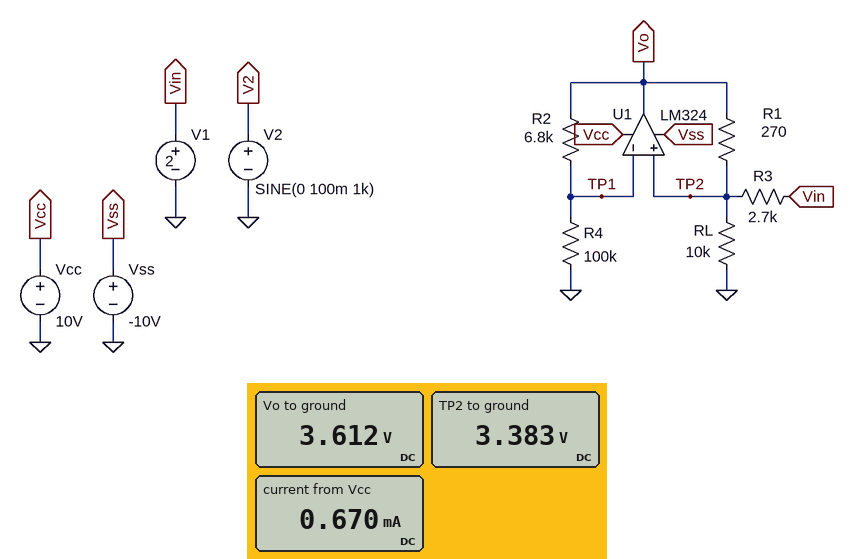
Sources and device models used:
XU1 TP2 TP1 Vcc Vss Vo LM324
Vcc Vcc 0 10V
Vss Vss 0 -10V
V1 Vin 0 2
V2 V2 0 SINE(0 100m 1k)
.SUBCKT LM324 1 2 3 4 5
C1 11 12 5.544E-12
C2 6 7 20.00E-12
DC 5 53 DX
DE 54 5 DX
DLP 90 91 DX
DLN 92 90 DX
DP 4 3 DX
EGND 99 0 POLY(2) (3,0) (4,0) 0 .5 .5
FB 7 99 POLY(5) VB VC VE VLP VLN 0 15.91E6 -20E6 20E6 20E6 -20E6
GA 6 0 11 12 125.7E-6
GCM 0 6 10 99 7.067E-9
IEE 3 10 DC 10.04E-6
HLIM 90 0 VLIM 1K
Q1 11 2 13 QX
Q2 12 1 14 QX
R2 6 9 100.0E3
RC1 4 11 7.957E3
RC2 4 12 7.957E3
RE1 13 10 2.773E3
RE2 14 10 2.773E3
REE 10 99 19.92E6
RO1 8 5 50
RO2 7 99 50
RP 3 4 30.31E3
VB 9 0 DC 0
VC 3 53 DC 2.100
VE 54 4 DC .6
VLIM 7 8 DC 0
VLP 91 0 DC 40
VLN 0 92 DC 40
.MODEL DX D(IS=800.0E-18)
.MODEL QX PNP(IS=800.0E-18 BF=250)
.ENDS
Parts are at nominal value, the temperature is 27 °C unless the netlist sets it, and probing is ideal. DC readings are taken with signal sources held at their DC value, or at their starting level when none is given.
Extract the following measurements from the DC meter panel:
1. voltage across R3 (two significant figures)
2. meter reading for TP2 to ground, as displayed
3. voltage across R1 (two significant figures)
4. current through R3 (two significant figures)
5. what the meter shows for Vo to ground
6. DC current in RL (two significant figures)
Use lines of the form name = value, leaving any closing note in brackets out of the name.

voltage across R3 = 1.4 V
meter reading for TP2 to ground, as displayed = 3.383 V
voltage across R1 = 230 mV
current through R3 = 510 µA
what the meter shows for Vo to ground = 3.612 V
DC current in RL = 340 µA
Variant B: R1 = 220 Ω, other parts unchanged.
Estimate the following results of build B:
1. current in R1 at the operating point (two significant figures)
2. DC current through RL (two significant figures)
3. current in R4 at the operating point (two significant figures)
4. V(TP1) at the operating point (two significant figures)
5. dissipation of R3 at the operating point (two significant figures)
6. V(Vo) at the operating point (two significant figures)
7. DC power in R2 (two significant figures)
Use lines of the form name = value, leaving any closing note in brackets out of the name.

current in R1 at the operating point = 1.4 mA
DC current through RL = 460 µA
current in R4 at the operating point = 46 µA
V(TP1) at the operating point = 4.6 V
dissipation of R3 at the operating point = 2.5 mW
V(Vo) at the operating point = 4.9 V
DC power in R2 = 14 µW
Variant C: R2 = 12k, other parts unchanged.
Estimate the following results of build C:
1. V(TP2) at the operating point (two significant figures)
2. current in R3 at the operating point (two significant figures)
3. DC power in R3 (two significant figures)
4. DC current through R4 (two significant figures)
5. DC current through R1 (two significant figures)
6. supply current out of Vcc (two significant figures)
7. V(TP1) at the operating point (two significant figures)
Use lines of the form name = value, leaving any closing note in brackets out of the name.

V(TP2) at the operating point = 7.7 V
current in R3 at the operating point = 2.1 mA
DC power in R3 = 12 mW
DC current through R4 = 76 µA
DC current through R1 = 2.9 mA
supply current out of Vcc = 660 µA
V(TP1) at the operating point = 7.6 V
